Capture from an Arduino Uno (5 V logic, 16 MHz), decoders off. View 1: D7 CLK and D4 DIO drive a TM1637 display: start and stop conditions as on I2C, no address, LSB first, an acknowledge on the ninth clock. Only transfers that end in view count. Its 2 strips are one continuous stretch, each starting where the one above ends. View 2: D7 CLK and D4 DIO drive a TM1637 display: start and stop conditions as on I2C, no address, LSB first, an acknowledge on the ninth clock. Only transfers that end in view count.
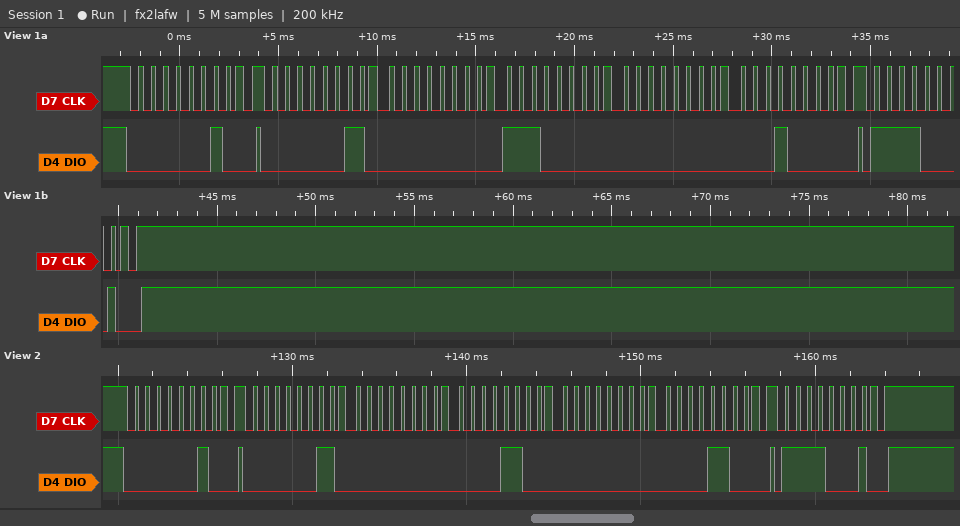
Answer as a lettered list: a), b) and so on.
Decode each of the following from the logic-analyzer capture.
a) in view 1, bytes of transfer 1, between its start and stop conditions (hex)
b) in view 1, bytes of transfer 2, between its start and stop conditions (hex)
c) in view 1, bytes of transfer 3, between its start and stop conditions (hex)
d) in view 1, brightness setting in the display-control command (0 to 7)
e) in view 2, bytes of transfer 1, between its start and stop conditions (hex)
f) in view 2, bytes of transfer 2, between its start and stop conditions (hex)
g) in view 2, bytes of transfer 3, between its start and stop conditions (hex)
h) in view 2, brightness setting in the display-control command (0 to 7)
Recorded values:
a) 40
b) C0 00 07 00 08
c) 8F
d) 7
e) 40
f) C0 00 30 00 30
g) 8F
h) 7
